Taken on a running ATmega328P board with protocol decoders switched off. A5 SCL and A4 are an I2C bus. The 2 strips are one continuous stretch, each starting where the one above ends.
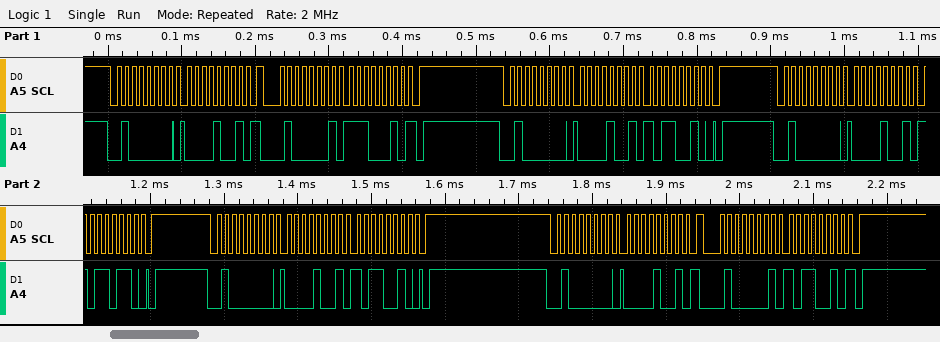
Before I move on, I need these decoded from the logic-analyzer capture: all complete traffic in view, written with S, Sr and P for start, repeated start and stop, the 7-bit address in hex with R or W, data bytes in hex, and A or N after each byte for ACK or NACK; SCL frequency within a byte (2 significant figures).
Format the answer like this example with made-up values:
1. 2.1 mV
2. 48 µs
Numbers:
1. S 20W A 09 A Sr 20R A E2 N P S 20W A 09 A B2 A P S 20W A 09 A B6 A P S 20W A 09 A B2 A P S 20W A 09 A Sr 20R A B2 N P
2. 100 kHz
